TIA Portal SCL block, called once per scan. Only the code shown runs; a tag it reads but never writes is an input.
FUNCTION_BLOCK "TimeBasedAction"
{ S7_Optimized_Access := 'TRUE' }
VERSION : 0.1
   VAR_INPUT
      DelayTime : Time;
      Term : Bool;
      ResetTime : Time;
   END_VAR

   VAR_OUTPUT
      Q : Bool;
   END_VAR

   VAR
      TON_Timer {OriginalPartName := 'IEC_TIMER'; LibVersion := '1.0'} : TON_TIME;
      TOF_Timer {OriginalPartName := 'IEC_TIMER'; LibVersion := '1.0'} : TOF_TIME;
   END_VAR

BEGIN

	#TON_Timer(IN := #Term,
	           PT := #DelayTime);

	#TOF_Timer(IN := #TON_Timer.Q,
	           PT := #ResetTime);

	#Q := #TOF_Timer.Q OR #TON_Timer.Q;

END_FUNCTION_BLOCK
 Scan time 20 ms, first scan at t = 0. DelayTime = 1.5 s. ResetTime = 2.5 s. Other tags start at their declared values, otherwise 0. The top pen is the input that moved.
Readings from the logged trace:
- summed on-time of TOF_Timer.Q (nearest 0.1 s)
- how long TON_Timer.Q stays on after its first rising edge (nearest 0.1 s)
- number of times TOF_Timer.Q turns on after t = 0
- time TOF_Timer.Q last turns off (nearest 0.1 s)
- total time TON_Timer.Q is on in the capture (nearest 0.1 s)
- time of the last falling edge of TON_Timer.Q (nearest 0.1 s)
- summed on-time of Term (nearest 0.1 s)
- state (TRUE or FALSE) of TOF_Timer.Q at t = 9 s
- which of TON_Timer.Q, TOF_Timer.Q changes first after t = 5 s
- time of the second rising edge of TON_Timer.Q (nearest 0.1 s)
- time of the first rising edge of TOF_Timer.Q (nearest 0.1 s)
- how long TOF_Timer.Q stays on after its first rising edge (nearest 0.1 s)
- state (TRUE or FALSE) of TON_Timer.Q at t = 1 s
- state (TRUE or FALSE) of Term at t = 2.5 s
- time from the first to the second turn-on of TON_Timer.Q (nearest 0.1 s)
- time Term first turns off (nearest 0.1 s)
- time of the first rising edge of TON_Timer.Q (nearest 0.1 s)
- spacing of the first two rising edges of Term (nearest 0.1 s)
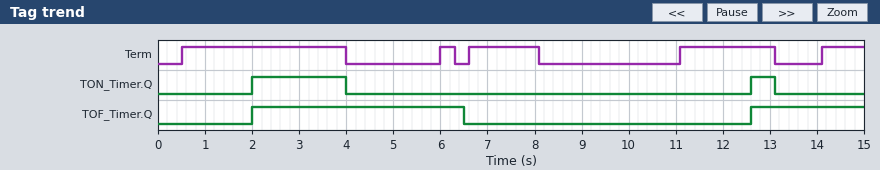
6.9 s
2.0 s
2
6.5 s
2.5 s
13.1 s
8.2 s
FALSE
TOF_Timer.Q
12.6 s
2.0 s
4.5 s
FALSE
TRUE
10.6 s
4.0 s
2.0 s
5.5 s
